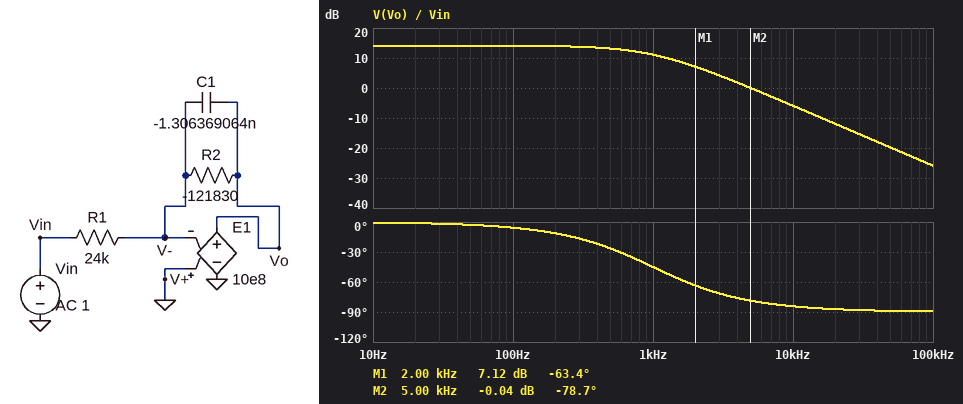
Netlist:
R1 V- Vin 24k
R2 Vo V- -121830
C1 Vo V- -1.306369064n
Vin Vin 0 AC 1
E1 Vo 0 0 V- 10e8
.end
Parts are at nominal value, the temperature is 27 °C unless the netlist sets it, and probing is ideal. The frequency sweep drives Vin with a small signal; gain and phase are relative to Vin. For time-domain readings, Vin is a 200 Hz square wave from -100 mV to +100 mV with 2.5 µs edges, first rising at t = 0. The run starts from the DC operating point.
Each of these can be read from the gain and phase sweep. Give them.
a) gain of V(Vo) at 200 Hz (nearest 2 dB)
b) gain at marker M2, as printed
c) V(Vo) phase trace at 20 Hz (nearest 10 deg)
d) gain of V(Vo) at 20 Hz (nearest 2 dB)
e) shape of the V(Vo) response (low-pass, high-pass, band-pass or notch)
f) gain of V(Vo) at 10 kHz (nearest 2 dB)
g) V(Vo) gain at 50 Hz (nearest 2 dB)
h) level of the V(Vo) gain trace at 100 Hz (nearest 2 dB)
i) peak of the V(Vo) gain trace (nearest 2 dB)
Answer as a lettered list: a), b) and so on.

a) 14 dB
b) -0.04 dB
c) 0 deg
d) 14 dB
e) low-pass
f) -6 dB
g) 14 dB
h) 14 dB
i) 14 dB
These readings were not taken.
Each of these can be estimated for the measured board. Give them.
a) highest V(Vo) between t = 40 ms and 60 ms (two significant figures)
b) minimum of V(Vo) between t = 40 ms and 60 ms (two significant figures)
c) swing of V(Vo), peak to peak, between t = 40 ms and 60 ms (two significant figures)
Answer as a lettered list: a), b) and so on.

a) 510 mV
b) -510 mV
c) 1.0 V
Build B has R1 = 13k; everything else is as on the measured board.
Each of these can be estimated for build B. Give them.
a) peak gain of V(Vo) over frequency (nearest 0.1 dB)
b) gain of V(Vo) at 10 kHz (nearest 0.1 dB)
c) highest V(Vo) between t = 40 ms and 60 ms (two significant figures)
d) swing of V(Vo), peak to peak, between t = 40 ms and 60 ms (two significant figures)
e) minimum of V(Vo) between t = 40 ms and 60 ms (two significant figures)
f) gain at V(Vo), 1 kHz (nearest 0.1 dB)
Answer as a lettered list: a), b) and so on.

a) 19.4 dB
b) -0.6 dB
c) 940 mV
d) 1.9 V
e) -940 mV
f) 16.4 dB
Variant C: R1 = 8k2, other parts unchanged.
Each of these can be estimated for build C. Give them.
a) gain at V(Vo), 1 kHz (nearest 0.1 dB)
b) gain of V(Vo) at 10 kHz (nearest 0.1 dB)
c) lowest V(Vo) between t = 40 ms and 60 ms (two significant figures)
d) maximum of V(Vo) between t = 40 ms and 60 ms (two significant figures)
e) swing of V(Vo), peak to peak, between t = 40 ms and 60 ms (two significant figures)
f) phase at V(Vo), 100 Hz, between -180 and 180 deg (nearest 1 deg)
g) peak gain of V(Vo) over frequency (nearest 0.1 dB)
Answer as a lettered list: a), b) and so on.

a) 20.4 dB
b) 3.4 dB
c) -1.5 V
d) 1.5 V
e) 3.0 V
f) -6 deg
g) 23.4 dB
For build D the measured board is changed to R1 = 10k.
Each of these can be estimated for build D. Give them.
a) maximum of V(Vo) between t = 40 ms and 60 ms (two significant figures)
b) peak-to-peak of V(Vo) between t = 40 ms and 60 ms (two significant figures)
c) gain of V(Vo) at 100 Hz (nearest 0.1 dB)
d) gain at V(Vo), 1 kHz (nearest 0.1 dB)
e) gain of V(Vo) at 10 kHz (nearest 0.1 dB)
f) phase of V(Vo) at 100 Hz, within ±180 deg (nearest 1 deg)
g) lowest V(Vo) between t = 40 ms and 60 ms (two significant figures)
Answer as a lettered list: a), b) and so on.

a) 1.2 V
b) 2.4 V
c) 21.7 dB
d) 18.7 dB
e) 1.7 dB
f) -6 deg
g) -1.2 V
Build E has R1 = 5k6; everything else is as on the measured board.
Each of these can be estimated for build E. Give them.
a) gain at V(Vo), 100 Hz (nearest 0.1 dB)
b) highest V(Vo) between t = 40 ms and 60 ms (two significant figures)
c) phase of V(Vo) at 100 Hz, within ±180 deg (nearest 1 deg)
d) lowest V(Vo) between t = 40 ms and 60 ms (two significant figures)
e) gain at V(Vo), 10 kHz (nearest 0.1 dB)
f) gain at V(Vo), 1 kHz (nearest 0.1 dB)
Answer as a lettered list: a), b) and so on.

a) 26.7 dB
b) 2.2 V
c) -6 deg
d) -2.2 V
e) 6.7 dB
f) 23.7 dB
